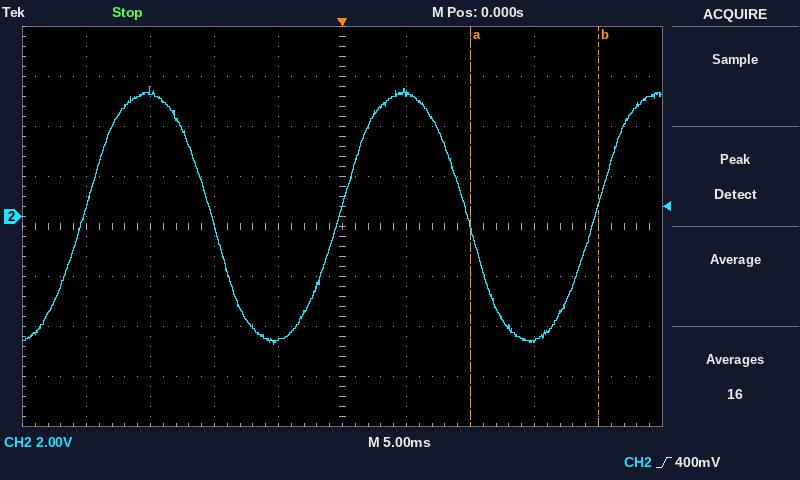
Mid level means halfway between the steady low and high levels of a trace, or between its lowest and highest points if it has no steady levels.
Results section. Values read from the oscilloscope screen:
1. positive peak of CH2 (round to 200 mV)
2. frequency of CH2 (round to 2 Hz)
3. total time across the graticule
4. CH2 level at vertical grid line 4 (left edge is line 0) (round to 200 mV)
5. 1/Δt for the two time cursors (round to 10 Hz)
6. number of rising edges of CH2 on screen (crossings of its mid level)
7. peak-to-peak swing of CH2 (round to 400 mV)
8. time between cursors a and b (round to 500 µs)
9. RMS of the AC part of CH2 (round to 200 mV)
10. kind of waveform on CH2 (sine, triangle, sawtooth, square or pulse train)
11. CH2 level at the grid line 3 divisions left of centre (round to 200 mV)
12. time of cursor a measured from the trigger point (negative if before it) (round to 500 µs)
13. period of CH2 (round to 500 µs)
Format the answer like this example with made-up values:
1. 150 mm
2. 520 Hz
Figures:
1. 5.2 V
2. 50 Hz
3. 50 ms
4. -5.0 V
5. 100 Hz
6. 3
7. 10.4 V
8. 10.0 ms
9. 3.6 V
10. sine
11. 5.0 V
12. +10.0 ms
13. 20.0 ms
